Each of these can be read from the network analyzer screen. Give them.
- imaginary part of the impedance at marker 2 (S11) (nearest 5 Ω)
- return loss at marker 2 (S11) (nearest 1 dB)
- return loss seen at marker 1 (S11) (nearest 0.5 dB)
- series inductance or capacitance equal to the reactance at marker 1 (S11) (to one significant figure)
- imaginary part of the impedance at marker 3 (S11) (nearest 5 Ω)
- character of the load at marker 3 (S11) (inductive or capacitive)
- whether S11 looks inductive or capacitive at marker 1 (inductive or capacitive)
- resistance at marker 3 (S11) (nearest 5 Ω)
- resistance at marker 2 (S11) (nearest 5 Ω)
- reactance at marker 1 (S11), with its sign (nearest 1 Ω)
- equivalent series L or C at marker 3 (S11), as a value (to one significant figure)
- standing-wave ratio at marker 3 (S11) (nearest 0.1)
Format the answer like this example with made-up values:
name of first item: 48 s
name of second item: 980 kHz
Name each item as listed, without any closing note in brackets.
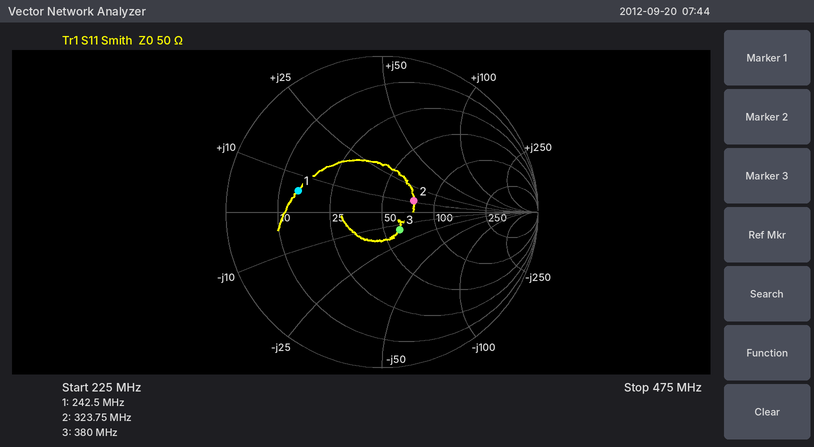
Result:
imaginary part of the impedance at marker 2 (S11): +10 Ω
return loss at marker 2 (S11): 13 dB
return loss seen at marker 1 (S11): 5.0 dB
series inductance or capacitance equal to the reactance at marker 1 (S11): 4 nH
imaginary part of the impedance at marker 3 (S11): -15 Ω
character of the load at marker 3 (S11): capacitive
whether S11 looks inductive or capacitive at marker 1: inductive
resistance at marker 3 (S11): 60 Ω
resistance at marker 2 (S11): 75 Ω
reactance at marker 1 (S11), with its sign: +6 Ω
equivalent series L or C at marker 3 (S11), as a value: 30 pF
standing-wave ratio at marker 3 (S11): 1.4
